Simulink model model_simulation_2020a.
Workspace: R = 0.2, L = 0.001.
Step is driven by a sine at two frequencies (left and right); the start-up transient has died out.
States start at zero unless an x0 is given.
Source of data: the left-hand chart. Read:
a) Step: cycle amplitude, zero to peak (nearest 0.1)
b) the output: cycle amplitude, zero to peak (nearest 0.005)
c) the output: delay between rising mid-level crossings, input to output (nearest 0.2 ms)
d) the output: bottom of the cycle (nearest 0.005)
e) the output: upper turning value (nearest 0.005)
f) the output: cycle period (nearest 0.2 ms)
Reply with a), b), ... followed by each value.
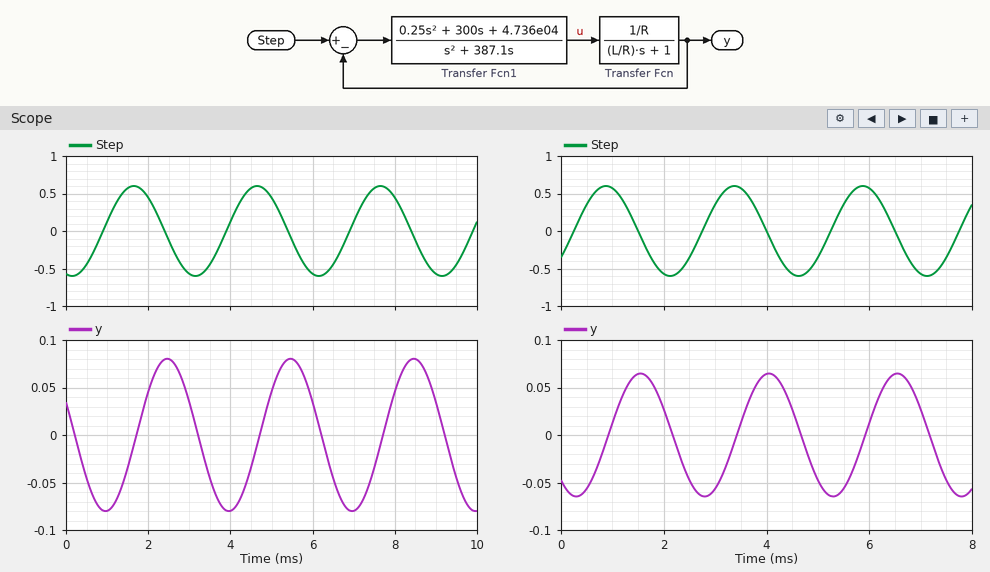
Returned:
a) 0.6
b) 0.080
c) 0.8 ms
d) -0.080
e) 0.080
f) 3.0 ms
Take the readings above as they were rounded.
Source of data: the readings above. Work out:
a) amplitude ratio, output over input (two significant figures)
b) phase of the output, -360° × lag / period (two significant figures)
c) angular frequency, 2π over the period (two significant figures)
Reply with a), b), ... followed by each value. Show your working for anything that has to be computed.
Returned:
a) 0.08 / 0.6 = 0.13
b) -360 × 0.8 / 3 = -96°
c) 2π / 3 = 2.1 rad/ms
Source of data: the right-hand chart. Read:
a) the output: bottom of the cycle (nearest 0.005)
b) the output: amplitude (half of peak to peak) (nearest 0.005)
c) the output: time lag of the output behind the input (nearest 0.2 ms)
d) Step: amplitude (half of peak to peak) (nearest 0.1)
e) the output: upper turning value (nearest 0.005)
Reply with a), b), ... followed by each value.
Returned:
a) -0.065
b) 0.065
c) 0.6 ms
d) 0.6
e) 0.065
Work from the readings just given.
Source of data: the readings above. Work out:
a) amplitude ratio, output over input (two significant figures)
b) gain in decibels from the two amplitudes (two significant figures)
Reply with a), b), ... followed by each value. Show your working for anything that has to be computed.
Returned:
a) 0.065 / 0.6 = 0.11
b) 20 log10(0.065 / 0.6) = -19 dB
